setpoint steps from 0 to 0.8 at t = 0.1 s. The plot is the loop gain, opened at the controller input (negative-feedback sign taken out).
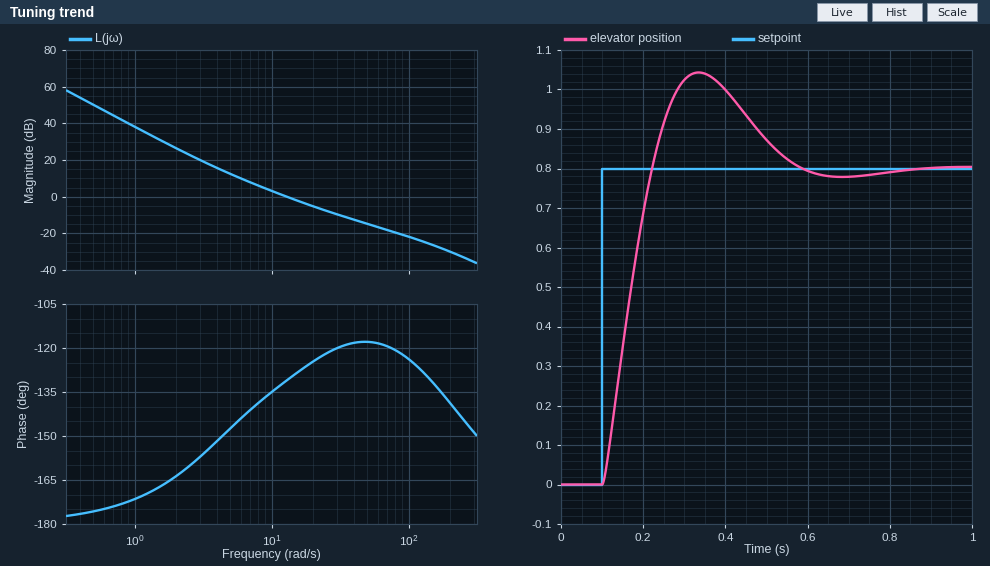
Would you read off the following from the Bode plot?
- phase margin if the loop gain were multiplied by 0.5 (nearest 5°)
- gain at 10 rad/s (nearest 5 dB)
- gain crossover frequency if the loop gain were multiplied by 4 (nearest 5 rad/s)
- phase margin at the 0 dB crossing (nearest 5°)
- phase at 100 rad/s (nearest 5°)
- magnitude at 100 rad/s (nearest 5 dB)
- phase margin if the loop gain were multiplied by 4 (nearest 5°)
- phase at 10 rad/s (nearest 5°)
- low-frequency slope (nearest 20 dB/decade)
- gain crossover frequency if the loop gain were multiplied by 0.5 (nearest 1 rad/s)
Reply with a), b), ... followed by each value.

a) 40°
b) 5 dB
c) 40 rad/s
d) 50°
e) -125°
f) -20 dB
g) 60°
h) -135°
i) -40 dB/decade
j) 8 rad/s
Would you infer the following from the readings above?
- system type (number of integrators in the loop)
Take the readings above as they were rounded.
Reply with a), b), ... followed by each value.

a) 2
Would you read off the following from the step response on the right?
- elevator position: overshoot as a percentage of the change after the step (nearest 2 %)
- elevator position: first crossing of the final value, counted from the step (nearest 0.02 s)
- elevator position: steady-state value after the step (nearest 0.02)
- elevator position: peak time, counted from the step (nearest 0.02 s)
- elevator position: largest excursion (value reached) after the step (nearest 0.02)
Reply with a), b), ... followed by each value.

a) 30 %
b) 0.12 s
c) 0.80
d) 0.24 s
e) 1.04
